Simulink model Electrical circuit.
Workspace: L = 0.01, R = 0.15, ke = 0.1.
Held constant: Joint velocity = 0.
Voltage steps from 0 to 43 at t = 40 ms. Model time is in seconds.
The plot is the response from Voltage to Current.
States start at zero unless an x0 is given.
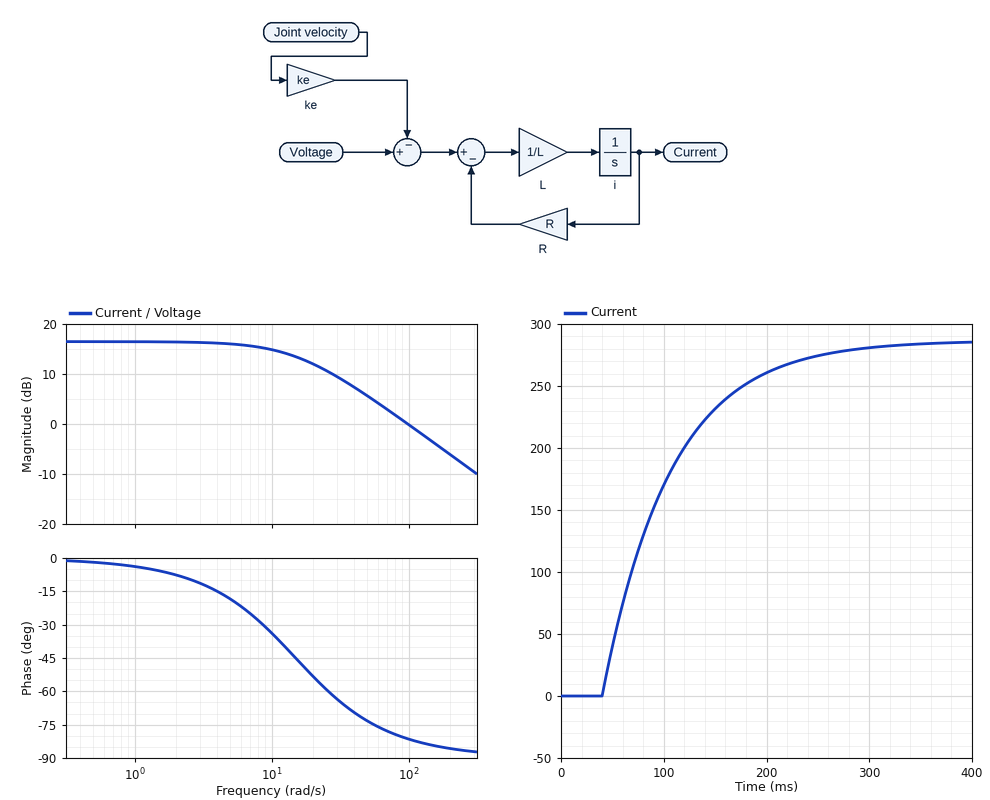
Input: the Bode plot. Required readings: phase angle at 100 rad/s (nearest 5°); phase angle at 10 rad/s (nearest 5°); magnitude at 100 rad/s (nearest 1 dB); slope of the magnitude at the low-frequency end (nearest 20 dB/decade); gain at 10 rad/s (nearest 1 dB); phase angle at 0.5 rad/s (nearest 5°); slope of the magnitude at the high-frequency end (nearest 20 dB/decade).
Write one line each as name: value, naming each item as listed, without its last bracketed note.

phase angle at 100 rad/s: -80°
phase angle at 10 rad/s: -35°
magnitude at 100 rad/s: 0 dB
slope of the magnitude at the low-frequency end: 0 dB/decade
gain at 10 rad/s: 15 dB
phase angle at 0.5 rad/s: 0°
slope of the magnitude at the high-frequency end: -20 dB/decade
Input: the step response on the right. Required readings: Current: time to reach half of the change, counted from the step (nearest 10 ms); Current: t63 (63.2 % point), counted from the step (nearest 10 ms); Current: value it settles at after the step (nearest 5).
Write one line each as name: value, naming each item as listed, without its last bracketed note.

Current: time to reach half of the change, counted from the step: 50 ms
Current: t63 (63.2 % point), counted from the step: 70 ms
Current: value it settles at after the step: 285
